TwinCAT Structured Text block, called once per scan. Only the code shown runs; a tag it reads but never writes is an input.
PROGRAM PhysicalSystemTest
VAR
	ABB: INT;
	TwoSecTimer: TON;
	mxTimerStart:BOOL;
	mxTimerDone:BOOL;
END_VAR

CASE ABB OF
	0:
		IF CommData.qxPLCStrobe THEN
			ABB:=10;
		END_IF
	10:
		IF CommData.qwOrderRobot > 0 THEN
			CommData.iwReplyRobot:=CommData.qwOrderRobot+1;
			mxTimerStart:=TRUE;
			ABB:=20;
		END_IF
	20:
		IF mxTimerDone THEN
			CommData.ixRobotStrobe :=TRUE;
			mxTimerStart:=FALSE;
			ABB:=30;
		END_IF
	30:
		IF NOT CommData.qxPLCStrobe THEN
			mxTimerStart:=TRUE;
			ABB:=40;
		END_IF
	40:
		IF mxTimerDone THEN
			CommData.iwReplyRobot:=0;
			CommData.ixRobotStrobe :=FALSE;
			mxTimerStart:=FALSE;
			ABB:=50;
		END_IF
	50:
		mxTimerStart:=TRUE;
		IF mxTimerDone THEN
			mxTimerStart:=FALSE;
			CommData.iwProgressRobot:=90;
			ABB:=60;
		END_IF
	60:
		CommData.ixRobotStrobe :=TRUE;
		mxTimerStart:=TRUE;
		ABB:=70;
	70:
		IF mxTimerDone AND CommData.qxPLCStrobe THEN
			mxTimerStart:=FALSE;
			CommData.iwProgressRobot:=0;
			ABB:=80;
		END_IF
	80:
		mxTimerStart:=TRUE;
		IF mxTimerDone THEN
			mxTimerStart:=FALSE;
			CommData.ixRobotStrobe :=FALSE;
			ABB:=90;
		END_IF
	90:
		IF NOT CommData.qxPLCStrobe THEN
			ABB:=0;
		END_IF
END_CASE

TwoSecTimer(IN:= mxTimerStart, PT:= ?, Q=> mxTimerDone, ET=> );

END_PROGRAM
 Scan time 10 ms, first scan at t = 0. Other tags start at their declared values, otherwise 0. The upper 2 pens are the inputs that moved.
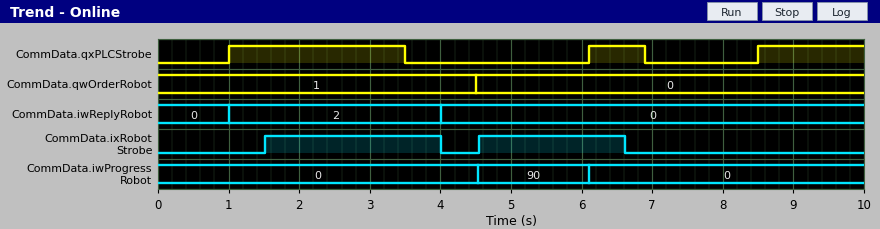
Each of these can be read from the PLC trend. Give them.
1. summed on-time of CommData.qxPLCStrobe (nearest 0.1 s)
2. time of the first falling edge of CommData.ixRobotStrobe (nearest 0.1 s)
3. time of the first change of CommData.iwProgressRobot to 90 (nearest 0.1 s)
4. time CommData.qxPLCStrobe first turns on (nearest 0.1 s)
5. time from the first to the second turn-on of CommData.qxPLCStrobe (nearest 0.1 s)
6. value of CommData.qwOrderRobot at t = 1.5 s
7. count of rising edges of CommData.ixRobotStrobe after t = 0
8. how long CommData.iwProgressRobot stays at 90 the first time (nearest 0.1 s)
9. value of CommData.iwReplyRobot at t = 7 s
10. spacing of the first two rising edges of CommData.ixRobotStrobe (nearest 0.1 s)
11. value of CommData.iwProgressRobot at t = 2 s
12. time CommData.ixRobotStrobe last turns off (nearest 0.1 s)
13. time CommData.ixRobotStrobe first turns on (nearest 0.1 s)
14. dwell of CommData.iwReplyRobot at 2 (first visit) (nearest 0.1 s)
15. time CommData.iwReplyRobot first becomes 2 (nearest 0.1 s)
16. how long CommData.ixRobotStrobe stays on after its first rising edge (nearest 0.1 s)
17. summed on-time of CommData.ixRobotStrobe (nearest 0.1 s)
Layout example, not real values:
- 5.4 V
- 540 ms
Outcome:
- 4.8 s
- 4.0 s
- 4.5 s
- 1.0 s
- 5.1 s
- 1
- 2
- 1.6 s
- 0
- 3.0 s
- 0
- 6.6 s
- 1.5 s
- 3.0 s
- 1.0 s
- 2.5 s
- 4.6 s
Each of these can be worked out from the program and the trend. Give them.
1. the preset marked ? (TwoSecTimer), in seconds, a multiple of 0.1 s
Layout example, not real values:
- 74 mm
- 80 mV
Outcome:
- 0.5 s
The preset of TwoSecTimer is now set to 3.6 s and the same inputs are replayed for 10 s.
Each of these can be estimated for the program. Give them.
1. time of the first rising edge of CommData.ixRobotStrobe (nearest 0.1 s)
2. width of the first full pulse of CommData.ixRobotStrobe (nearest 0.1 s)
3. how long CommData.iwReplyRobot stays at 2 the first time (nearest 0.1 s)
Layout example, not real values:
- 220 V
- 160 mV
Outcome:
- 4.6 s
- 3.6 s
- 7.2 s
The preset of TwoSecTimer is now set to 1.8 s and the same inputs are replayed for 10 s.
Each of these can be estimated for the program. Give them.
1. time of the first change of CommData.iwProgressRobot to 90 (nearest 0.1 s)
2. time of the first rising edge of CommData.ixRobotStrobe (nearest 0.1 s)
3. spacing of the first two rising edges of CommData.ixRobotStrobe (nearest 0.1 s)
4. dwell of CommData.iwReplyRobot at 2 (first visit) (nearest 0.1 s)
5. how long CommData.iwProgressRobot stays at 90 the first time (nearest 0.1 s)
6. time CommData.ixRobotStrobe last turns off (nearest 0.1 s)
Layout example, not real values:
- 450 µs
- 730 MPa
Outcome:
- 7.1 s
- 2.8 s
- 4.3 s
- 4.3 s
- 1.8 s
- 5.3 s
